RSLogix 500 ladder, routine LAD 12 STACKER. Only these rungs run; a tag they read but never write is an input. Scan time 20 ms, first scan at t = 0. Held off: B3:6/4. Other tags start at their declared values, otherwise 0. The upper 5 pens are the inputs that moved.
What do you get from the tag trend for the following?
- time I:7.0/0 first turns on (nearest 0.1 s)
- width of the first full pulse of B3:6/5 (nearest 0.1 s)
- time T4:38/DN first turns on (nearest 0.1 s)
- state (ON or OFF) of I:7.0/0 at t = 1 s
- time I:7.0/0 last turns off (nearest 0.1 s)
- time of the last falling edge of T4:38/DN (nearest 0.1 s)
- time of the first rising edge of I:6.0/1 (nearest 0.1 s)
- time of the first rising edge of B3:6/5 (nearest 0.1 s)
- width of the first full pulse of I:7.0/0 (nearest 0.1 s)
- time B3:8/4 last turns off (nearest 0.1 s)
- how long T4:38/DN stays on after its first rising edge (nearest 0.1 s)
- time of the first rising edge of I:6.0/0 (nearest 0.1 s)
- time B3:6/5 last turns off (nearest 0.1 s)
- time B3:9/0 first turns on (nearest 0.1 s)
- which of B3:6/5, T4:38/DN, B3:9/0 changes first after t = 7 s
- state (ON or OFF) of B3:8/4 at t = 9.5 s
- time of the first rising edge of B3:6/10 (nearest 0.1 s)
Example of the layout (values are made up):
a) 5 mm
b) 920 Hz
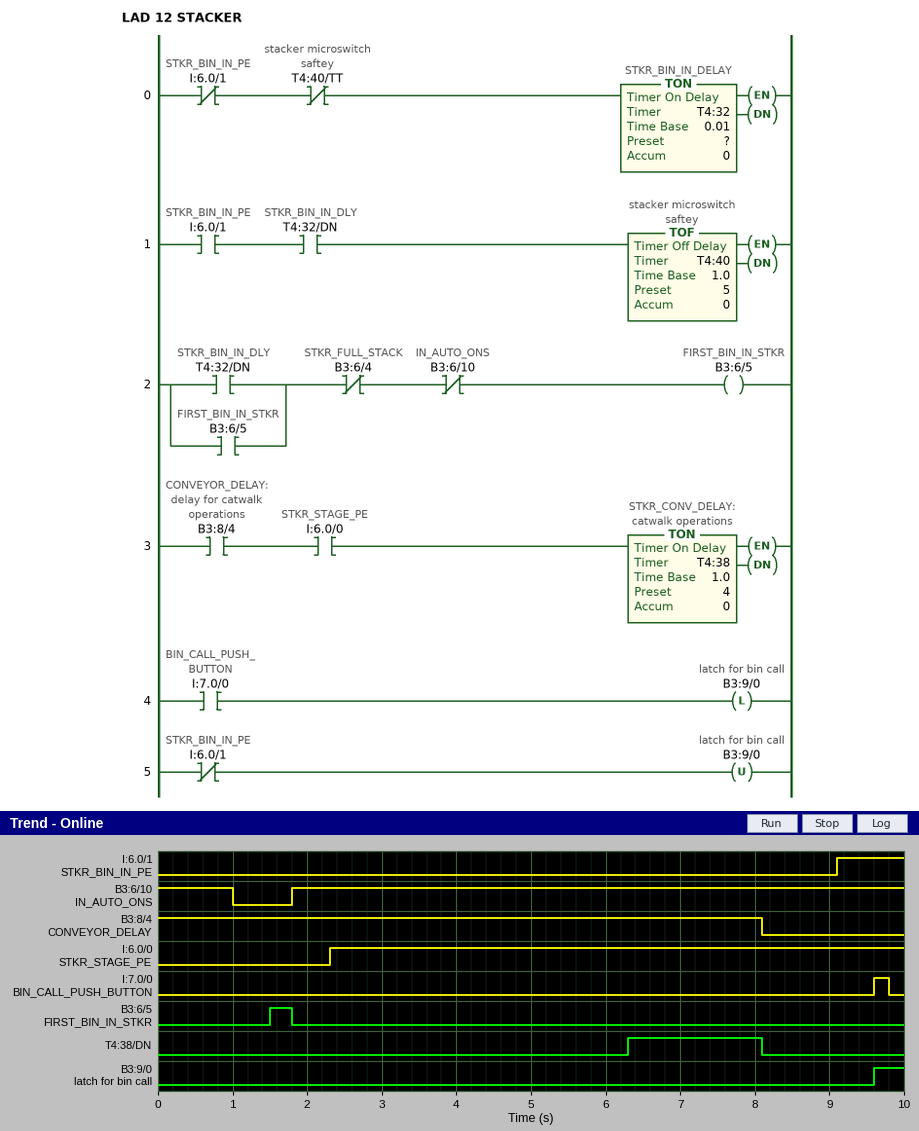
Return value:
a) 9.6 s
b) 0.3 s
c) 6.3 s
d) OFF
e) 9.8 s
f) 8.1 s
g) 9.1 s
h) 1.5 s
i) 0.2 s
j) 8.1 s
k) 1.8 s
l) 2.3 s
m) 1.8 s
n) 9.6 s
o) T4:38/DN
p) OFF
q) 1.8 s
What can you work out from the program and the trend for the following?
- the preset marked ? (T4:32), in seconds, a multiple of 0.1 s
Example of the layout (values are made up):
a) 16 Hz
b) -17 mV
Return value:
a) 1.5 s
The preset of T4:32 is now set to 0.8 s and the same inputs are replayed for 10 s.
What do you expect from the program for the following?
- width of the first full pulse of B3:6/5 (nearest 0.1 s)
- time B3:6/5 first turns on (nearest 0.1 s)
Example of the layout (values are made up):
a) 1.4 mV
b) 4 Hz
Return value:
a) 0.8 s
b) 1.0 s
